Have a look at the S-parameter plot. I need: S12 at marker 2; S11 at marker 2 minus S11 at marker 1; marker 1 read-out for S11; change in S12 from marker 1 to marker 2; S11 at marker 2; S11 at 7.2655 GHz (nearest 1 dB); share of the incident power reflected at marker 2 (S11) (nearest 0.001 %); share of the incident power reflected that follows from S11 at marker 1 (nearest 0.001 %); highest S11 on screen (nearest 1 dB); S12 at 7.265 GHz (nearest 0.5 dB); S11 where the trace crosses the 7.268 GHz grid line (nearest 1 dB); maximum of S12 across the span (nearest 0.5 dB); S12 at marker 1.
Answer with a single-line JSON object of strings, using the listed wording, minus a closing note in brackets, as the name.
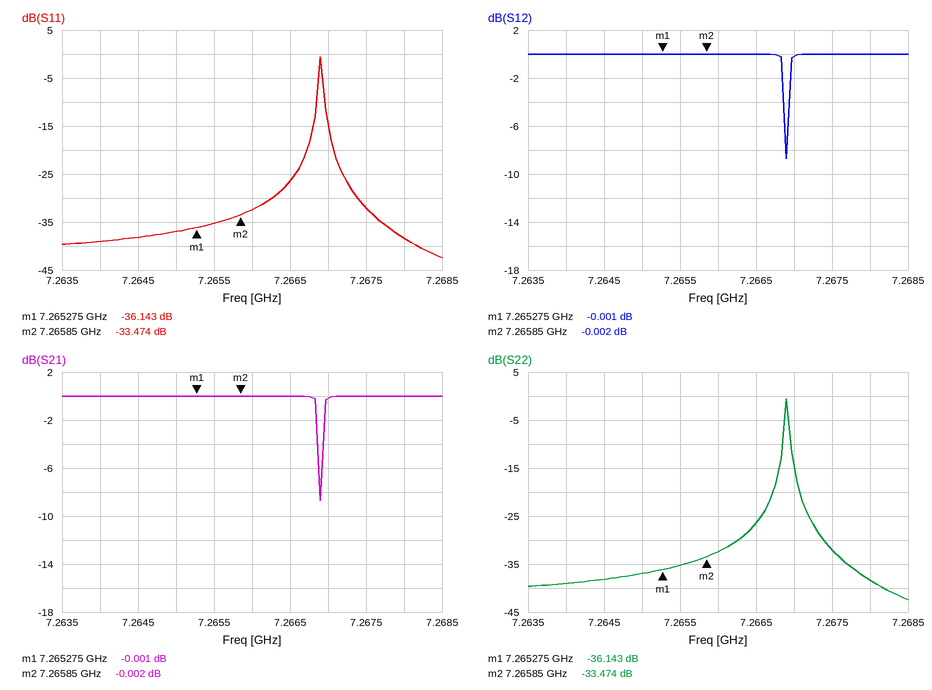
{"S12 at marker 2": "-0.002 dB", "S11 at marker 2 minus S11 at marker 1": "2.669 dB", "marker 1 read-out for S11": "-36.143 dB", "change in S12 from marker 1 to marker 2": "-0.001 dB", "S11 at marker 2": "-33.474 dB", "S11 at 7.2655 GHz": "-35 dB", "share of the incident power reflected at marker 2 (S11)": "0.045 %", "share of the incident power reflected that follows from S11 at marker 1": "0.024 %", "highest S11 on screen": "-1 dB", "S12 at 7.265 GHz": "0.0 dB", "S11 where the trace crosses the 7.268 GHz grid line": "-38 dB", "maximum of S12 across the span": "0.0 dB", "S12 at marker 1": "-0.001 dB"}
